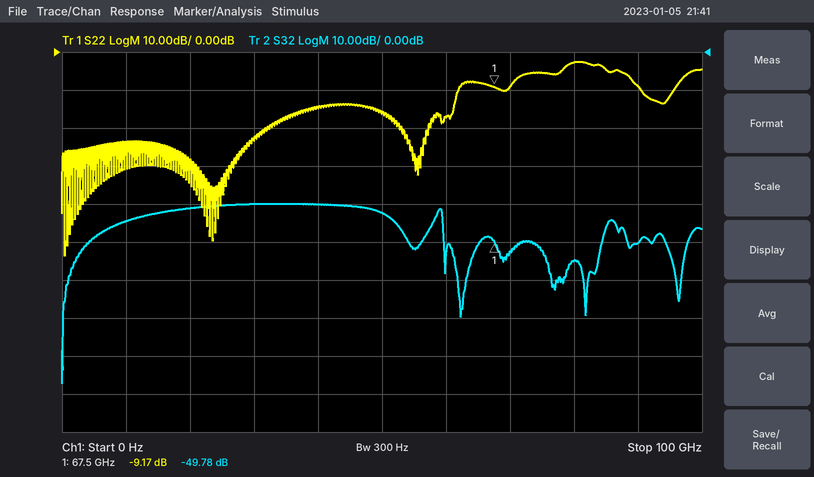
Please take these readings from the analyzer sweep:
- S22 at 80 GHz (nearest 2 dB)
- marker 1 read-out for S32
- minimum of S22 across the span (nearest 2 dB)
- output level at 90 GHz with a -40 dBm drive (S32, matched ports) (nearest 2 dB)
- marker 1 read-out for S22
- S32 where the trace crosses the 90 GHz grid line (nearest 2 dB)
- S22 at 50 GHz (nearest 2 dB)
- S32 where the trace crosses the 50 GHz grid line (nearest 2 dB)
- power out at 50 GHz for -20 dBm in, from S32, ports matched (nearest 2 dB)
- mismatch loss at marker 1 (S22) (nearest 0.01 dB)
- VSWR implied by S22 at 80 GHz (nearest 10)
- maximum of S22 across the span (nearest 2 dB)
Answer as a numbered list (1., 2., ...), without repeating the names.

1. -2 dB
2. -49.78 dB
3. -54 dB
4. -90 dBm
5. -9.17 dB
6. -50 dB
7. -16 dB
8. -42 dB
9. -62 dBm
10. 0.56 dB
11. 10
12. -2 dB
